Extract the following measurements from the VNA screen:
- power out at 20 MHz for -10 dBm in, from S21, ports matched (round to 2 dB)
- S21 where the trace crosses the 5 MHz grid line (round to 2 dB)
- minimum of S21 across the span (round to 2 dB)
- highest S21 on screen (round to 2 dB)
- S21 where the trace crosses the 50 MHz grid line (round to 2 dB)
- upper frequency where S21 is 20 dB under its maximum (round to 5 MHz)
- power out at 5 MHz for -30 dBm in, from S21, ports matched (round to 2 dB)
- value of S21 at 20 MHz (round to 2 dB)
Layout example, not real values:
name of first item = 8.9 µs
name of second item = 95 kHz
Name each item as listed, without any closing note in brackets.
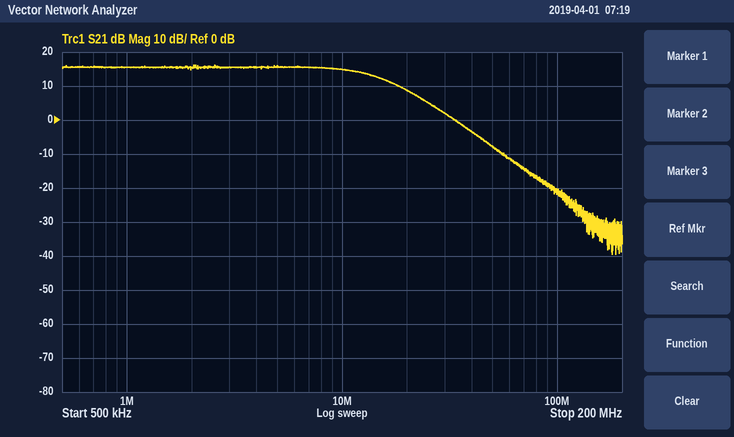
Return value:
power out at 20 MHz for -10 dBm in, from S21, ports matched = -2 dBm
S21 where the trace crosses the 5 MHz grid line = 16 dB
minimum of S21 across the span = -40 dB
highest S21 on screen = 16 dB
S21 where the trace crosses the 50 MHz grid line = -8 dB
upper frequency where S21 is 20 dB under its maximum = 40 MHz
power out at 5 MHz for -30 dBm in, from S21, ports matched = -14 dBm
value of S21 at 20 MHz = 8 dB
